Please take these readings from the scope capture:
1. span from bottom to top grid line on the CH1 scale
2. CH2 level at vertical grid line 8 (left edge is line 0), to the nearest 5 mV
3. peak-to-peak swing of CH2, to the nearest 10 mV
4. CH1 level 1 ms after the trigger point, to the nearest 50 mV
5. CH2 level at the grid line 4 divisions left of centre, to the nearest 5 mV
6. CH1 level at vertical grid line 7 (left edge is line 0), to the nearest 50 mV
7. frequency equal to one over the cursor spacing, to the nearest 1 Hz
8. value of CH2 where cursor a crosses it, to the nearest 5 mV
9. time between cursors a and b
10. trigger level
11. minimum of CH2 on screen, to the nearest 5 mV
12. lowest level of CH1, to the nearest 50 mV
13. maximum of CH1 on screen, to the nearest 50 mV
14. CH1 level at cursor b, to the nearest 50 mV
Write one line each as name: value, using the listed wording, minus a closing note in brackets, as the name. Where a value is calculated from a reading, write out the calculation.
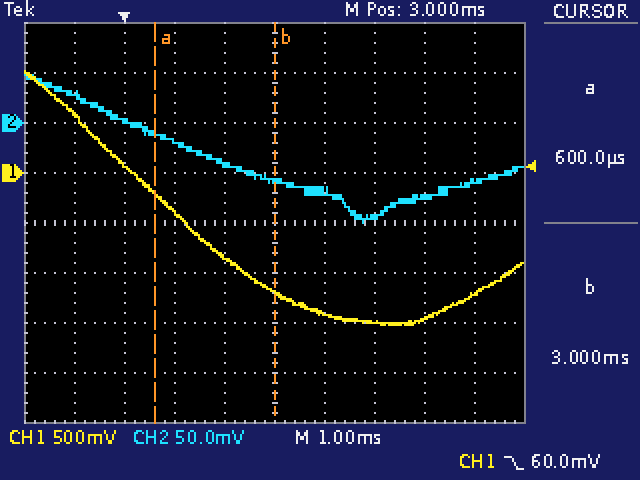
span from bottom to top grid line on the CH1 scale: 4 V
CH2 level at vertical grid line 8 (left edge is line 0), to the nearest 5 mV: -75 mV
peak-to-peak swing of CH2, to the nearest 10 mV: 150 mV
CH1 level 1 ms after the trigger point, to the nearest 50 mV: -400 mV
CH2 level at the grid line 4 divisions left of centre, to the nearest 5 mV: 30 mV
CH1 level at vertical grid line 7 (left edge is line 0), to the nearest 50 mV: -1.50 V
frequency equal to one over the cursor spacing, to the nearest 1 Hz: 1 / 2.4 ms ≈ 417 Hz
value of CH2 where cursor a crosses it, to the nearest 5 mV: -10 mV
time between cursors a and b: 3 ms − (600 µs) = 2.4 ms
trigger level: 60.0 mV
minimum of CH2 on screen, to the nearest 5 mV: -100 mV
lowest level of CH1, to the nearest 50 mV: -1.50 V
maximum of CH1 on screen, to the nearest 50 mV: 1.00 V
CH1 level at cursor b, to the nearest 50 mV: -1.20 V
